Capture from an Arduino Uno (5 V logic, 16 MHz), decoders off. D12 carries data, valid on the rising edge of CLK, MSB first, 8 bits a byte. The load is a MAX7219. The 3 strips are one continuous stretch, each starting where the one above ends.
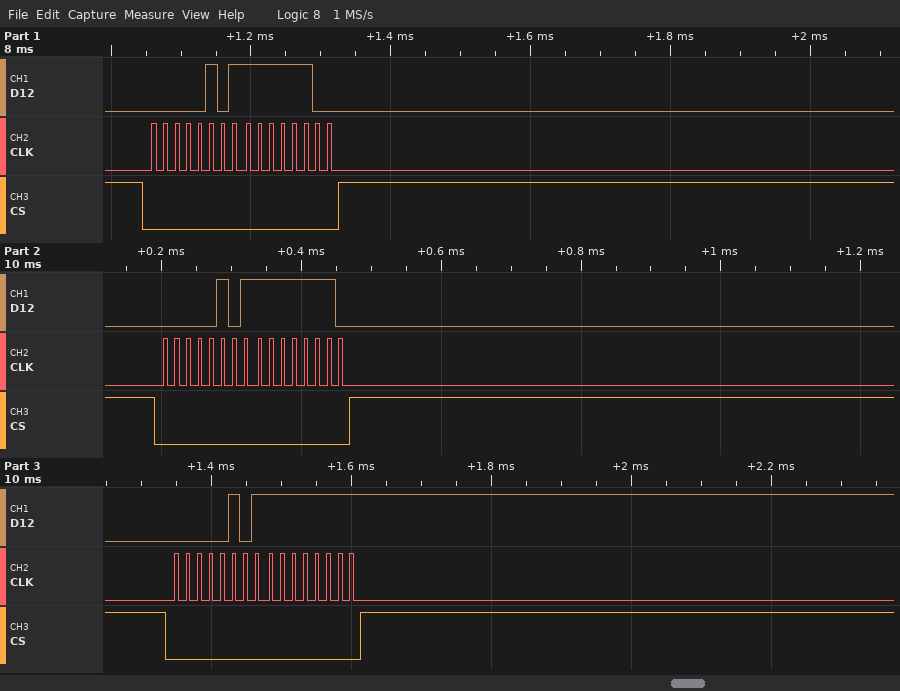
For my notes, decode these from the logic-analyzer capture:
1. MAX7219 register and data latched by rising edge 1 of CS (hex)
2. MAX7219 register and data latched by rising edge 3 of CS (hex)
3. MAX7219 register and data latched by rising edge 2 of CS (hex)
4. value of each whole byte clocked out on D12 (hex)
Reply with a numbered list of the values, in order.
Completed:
1. register 0x5, data 0xFC
2. register 0x5, data 0xFF
3. register 0x5, data 0xFE
4. 05 FC 05 FE 05 FF
